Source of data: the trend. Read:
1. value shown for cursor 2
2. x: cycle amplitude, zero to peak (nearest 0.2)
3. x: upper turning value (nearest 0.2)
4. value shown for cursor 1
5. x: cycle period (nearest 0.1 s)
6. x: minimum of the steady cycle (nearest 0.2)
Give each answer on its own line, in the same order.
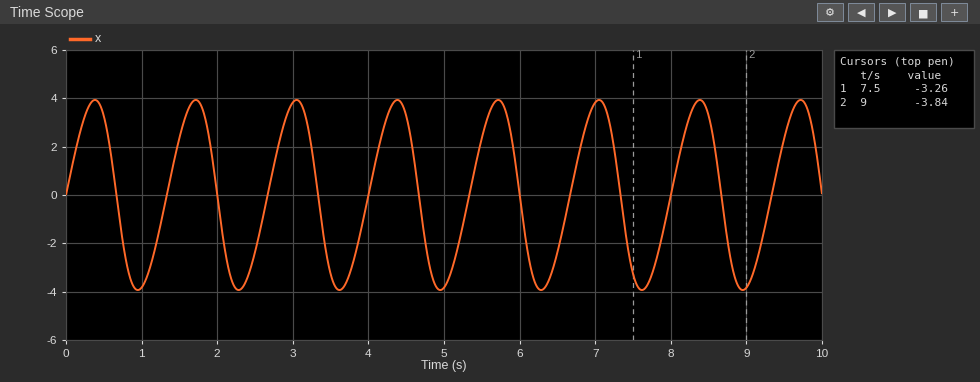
-3.84
4.0
4.0
-3.26
1.3 s
-4.0
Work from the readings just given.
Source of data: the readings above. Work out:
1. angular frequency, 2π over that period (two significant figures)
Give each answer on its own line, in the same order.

4.8 rad/s
